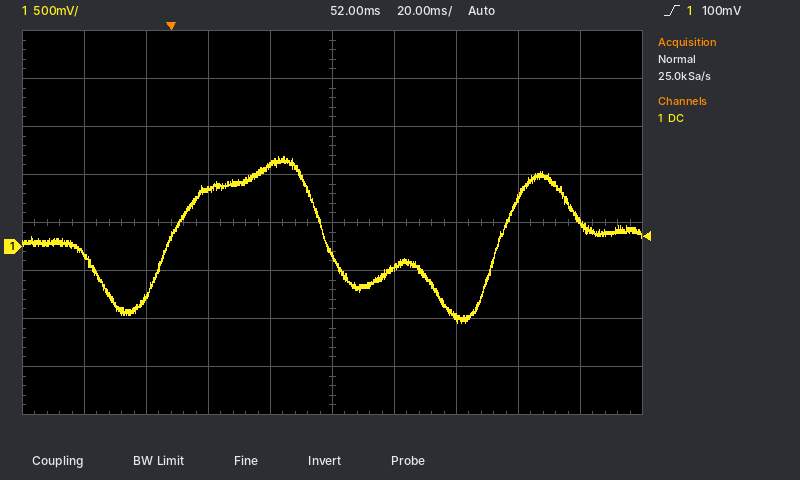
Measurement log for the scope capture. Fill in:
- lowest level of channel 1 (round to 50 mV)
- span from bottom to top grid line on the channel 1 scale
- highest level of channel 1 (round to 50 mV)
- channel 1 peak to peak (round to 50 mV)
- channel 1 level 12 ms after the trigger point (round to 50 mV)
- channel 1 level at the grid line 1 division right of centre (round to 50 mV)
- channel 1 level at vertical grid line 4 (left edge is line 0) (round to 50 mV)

-800 mV
4 V
950 mV
1.75 V
600 mV
-200 mV
850 mV
